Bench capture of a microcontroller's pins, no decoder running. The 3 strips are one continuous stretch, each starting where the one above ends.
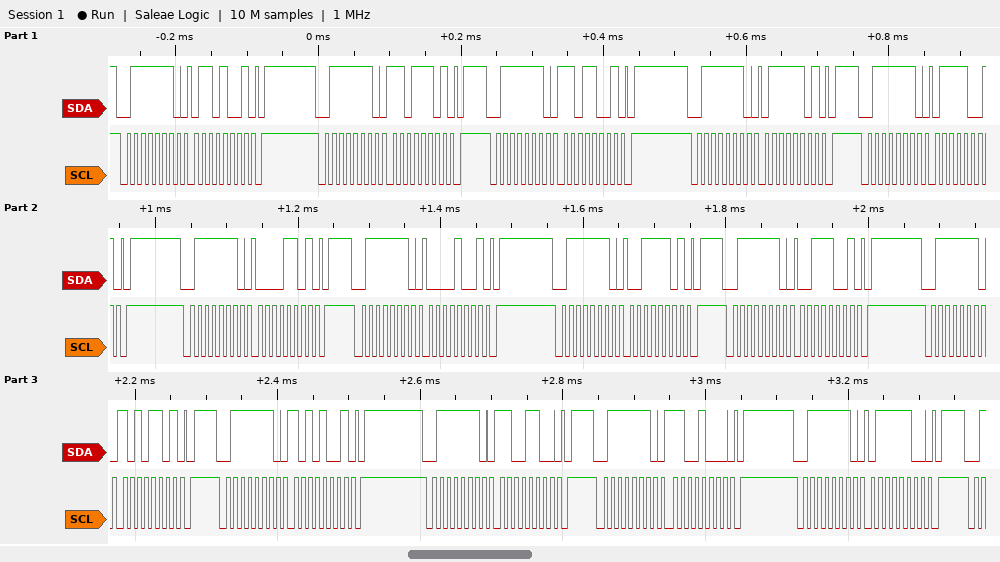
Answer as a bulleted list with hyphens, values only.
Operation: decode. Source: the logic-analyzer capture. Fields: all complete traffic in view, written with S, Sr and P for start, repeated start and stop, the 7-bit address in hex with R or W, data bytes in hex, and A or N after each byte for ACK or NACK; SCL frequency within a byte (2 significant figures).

- S 3FW A 69 A P S 3FW A DD A P S 3FW A D9 A P S 3FW A 7D A P S 3FW A 79 A P S 3FW A 0D A P S 3FW A 09 A P S 3FW A 3D A P S 3FW A 39 A P S 3FW A AD A P S 3FW A A9 A P S 3FW A CC A P S 3FW A C8 A P S 3FW A 7C A P
- 100 kHz
